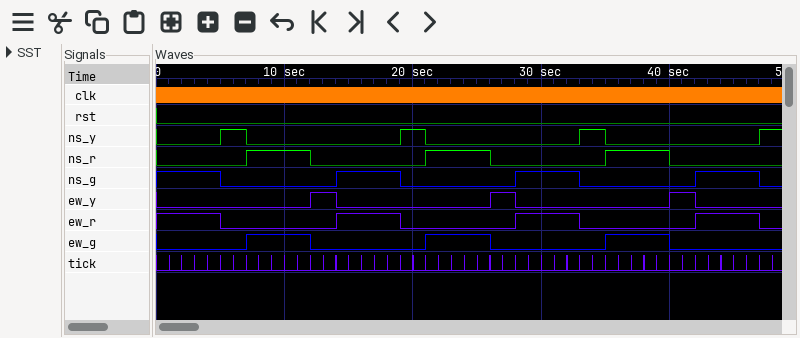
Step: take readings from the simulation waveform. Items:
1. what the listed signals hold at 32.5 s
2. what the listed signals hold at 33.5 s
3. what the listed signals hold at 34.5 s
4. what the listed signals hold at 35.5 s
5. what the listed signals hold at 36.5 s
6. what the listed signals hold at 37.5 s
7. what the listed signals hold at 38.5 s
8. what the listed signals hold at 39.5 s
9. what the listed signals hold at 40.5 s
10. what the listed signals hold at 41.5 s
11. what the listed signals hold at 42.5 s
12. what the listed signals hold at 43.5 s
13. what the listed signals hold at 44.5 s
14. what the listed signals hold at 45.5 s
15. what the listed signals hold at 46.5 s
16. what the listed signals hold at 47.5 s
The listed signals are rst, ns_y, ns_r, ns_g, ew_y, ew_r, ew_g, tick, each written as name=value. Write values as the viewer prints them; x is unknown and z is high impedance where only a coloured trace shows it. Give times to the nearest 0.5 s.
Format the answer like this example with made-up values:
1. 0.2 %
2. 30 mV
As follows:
1. rst=0, ns_y=0, ns_r=0, ns_g=1, ew_y=0, ew_r=1, ew_g=0, tick=0
2. rst=0, ns_y=1, ns_r=0, ns_g=0, ew_y=0, ew_r=0, ew_g=0, tick=0
3. rst=0, ns_y=1, ns_r=0, ns_g=0, ew_y=0, ew_r=0, ew_g=0, tick=0
4. rst=0, ns_y=0, ns_r=1, ns_g=0, ew_y=0, ew_r=0, ew_g=1, tick=0
5. rst=0, ns_y=0, ns_r=1, ns_g=0, ew_y=0, ew_r=0, ew_g=1, tick=0
6. rst=0, ns_y=0, ns_r=1, ns_g=0, ew_y=0, ew_r=0, ew_g=1, tick=0
7. rst=0, ns_y=0, ns_r=1, ns_g=0, ew_y=0, ew_r=0, ew_g=1, tick=0
8. rst=0, ns_y=0, ns_r=1, ns_g=0, ew_y=0, ew_r=0, ew_g=1, tick=0
9. rst=0, ns_y=0, ns_r=0, ns_g=0, ew_y=1, ew_r=0, ew_g=0, tick=0
10. rst=0, ns_y=0, ns_r=0, ns_g=0, ew_y=1, ew_r=0, ew_g=0, tick=0
11. rst=0, ns_y=0, ns_r=0, ns_g=1, ew_y=0, ew_r=1, ew_g=0, tick=0
12. rst=0, ns_y=0, ns_r=0, ns_g=1, ew_y=0, ew_r=1, ew_g=0, tick=0
13. rst=0, ns_y=0, ns_r=0, ns_g=1, ew_y=0, ew_r=1, ew_g=0, tick=0
14. rst=0, ns_y=0, ns_r=0, ns_g=1, ew_y=0, ew_r=1, ew_g=0, tick=0
15. rst=0, ns_y=0, ns_r=0, ns_g=1, ew_y=0, ew_r=1, ew_g=0, tick=0
16. rst=0, ns_y=1, ns_r=0, ns_g=0, ew_y=0, ew_r=0, ew_g=0, tick=0
